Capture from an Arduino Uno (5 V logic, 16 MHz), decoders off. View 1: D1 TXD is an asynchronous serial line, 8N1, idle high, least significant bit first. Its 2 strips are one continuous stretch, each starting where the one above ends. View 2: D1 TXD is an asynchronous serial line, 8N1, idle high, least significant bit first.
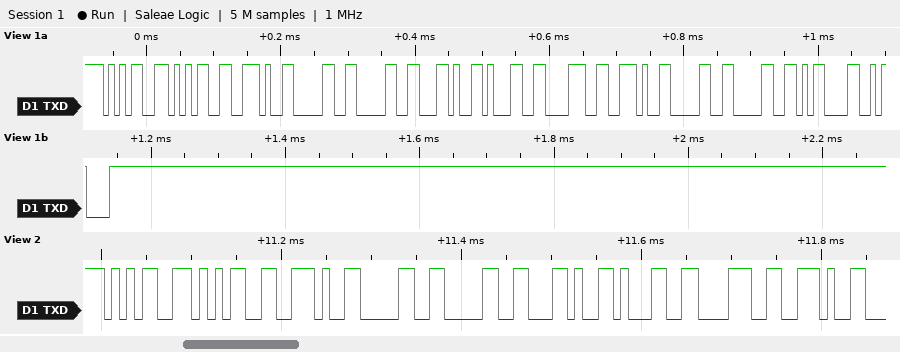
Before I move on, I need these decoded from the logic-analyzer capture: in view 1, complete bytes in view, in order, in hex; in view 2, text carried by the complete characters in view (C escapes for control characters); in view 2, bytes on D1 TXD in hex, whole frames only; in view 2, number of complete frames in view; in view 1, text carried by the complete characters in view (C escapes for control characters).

0x35 0x35 0x2E 0x30 0x30 0x2C 0x31 0x38 0x2E 0x30 0x30 0x0D 0x0A
"55.00,18."
35 35 2E 30 30 2C 31 38 2E
9
"55.00,18.00\r\n"
